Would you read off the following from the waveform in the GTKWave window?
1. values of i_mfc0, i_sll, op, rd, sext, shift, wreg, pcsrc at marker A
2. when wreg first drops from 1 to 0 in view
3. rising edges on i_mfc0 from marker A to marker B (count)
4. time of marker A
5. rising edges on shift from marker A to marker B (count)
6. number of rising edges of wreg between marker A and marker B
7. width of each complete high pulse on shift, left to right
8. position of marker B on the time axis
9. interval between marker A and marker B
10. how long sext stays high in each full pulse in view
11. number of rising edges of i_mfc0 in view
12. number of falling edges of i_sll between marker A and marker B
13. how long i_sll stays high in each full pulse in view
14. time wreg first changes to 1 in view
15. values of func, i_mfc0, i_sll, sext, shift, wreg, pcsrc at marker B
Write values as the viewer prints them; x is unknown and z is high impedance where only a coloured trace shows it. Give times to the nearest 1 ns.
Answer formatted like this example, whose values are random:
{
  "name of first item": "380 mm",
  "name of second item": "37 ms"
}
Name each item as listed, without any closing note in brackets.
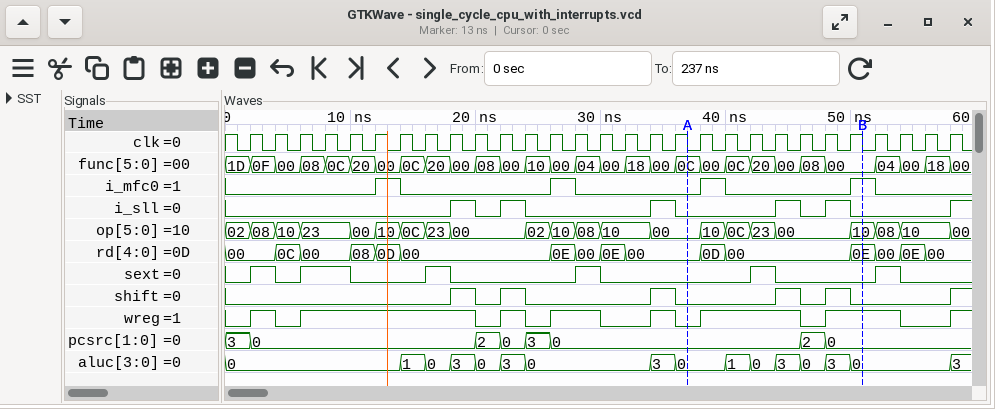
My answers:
{
  "values of i_mfc0, i_sll, op, rd, sext, shift, wreg, pcsrc at marker A": "i_mfc0=0, i_sll=0, op=00, rd=00, sext=0, shift=0, wreg=0, pcsrc=0",
  "when wreg first drops from 1 to 0 in view": "4 ns",
  "rising edges on i_mfc0 from marker A to marker B": "2",
  "time of marker A": "37 ns",
  "rising edges on shift from marker A to marker B": "2",
  "number of rising edges of wreg between marker A and marker B": "2",
  "width of each complete high pulse on shift, left to right": "2 ns, 2 ns, 2 ns, 2 ns, 2 ns",
  "position of marker B on the time axis": "51 ns",
  "interval between marker A and marker B": "14 ns",
  "how long sext stays high in each full pulse in view": "2 ns, 4 ns, 2 ns, 2 ns, 2 ns, 2 ns",
  "number of rising edges of i_mfc0 in view": "4",
  "number of falling edges of i_sll between marker A and marker B": "2",
  "how long i_sll stays high in each full pulse in view": "2 ns, 2 ns, 2 ns, 2 ns, 2 ns",
  "time wreg first changes to 1 in view": "2 ns",
  "values of func, i_mfc0, i_sll, sext, shift, wreg, pcsrc at marker B": "func=00, i_mfc0=1, i_sll=0, sext=0, shift=0, wreg=1, pcsrc=0"
}
